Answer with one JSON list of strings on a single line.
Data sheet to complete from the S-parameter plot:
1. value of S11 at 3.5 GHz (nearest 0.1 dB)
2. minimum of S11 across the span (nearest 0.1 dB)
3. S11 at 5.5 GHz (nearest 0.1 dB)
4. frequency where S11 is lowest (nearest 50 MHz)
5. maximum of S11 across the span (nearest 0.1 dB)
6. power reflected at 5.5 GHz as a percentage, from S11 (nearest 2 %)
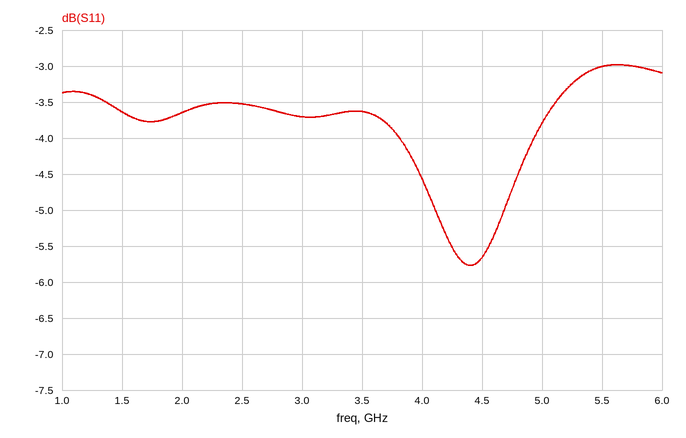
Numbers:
["-3.6 dB", "-5.8 dB", "-3.0 dB", "4.40 GHz", "-3.0 dB", "50 %"]
